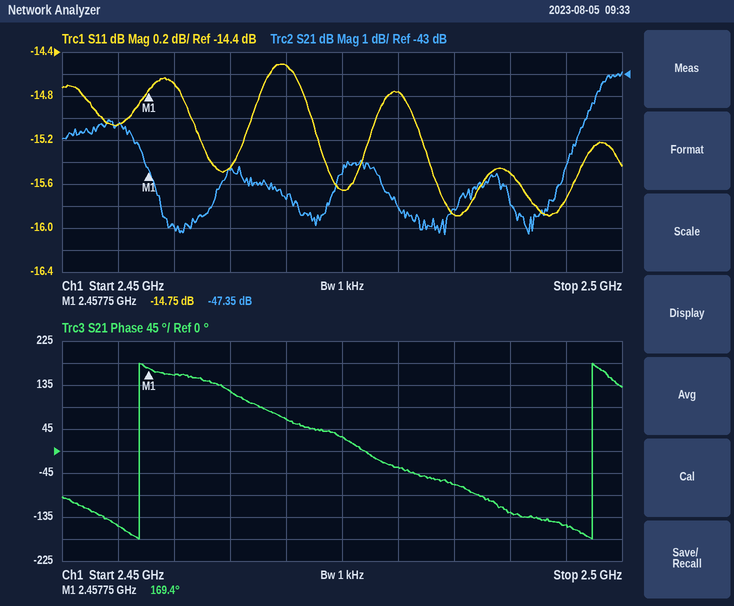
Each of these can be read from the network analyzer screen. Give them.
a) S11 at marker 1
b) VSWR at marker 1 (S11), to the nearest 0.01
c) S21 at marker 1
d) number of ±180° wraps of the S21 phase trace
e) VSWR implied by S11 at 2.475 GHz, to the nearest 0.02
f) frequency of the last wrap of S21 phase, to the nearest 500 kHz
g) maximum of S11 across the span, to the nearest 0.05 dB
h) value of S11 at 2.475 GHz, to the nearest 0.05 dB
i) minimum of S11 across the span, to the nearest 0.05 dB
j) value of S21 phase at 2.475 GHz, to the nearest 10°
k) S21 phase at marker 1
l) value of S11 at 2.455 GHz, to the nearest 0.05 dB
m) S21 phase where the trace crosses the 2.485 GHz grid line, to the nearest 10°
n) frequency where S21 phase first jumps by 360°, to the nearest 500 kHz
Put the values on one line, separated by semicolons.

-14.75 dB; 1.45; -47.35 dB; 2; 1.40; 2.4975 GHz; -14.50 dB; -15.65 dB; -15.90 dB; 30°; 169.4°; -15.05 dB; -70°; 2.4570 GHz
